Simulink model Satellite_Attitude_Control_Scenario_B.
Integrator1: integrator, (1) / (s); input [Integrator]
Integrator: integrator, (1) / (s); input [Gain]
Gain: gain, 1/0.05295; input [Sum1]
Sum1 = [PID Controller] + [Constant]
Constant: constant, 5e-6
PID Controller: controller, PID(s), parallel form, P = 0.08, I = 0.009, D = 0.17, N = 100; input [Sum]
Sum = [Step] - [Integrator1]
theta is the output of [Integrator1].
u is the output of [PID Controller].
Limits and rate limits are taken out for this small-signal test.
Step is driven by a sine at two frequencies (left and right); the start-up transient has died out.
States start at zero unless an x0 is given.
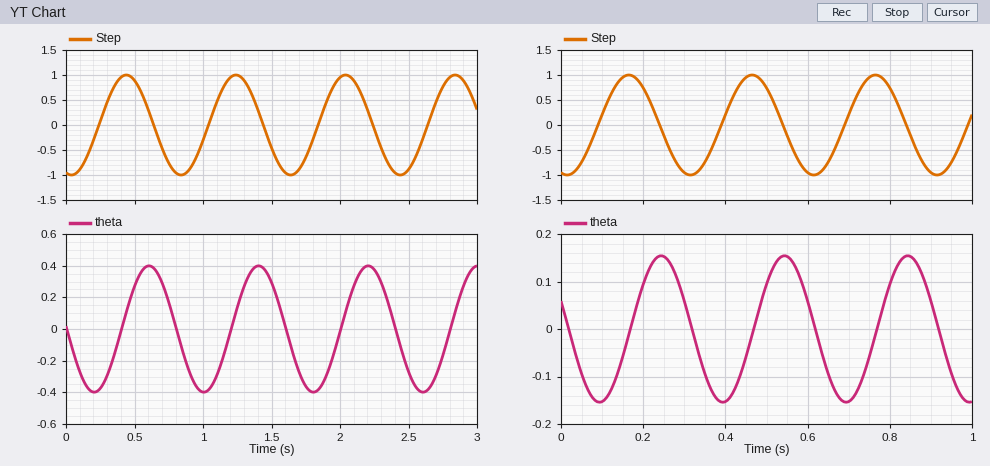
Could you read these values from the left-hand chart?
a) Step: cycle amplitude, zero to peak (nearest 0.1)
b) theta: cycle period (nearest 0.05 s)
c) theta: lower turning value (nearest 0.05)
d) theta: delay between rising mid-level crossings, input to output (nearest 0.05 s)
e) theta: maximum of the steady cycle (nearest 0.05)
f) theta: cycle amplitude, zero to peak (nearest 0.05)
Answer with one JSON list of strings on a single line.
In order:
["1.0", "0.80 s", "-0.40", "0.15 s", "0.40", "0.40"]
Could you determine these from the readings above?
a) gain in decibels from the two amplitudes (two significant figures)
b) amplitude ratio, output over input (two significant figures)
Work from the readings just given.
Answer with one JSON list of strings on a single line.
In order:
["-8.0 dB", "0.40"]
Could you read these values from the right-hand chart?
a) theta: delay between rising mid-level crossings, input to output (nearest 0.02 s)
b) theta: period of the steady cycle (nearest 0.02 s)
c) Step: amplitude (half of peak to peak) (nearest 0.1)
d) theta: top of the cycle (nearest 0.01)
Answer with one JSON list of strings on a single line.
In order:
["0.08 s", "0.30 s", "1.0", "0.15"]
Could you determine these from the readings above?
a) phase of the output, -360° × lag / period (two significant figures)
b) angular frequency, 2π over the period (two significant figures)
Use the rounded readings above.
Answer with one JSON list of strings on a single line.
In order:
["-96°", "21 rad/s"]
